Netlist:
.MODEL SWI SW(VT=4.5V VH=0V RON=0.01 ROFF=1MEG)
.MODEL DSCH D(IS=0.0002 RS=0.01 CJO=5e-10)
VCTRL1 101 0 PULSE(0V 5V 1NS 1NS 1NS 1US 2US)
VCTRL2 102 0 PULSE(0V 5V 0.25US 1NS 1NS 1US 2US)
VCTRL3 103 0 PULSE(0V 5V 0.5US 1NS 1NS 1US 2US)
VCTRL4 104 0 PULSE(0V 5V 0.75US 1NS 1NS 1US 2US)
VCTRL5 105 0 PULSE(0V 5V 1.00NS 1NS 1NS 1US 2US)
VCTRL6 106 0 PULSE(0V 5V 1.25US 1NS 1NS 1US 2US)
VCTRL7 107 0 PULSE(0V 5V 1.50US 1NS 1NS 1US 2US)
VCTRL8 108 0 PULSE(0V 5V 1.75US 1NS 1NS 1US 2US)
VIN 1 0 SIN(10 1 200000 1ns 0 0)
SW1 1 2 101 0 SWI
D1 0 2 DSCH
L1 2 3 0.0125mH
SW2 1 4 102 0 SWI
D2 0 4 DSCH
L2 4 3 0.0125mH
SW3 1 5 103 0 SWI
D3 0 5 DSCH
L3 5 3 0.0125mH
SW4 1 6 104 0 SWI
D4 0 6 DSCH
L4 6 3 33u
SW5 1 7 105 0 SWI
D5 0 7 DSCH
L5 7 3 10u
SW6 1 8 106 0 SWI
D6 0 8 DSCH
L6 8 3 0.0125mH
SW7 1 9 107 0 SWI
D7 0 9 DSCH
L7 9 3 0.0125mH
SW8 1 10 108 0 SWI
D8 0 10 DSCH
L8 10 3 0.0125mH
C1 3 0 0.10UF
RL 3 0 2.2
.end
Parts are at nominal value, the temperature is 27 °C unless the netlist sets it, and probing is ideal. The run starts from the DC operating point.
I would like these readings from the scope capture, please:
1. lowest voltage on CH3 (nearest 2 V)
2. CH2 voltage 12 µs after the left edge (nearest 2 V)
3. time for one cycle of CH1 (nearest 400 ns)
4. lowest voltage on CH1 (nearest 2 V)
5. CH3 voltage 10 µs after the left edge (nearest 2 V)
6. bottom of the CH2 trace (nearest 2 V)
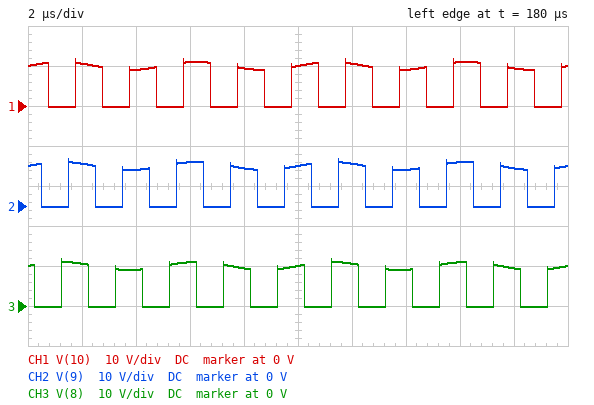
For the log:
0 V
10 V
2.0 µs
0 V
10 V
0 V
